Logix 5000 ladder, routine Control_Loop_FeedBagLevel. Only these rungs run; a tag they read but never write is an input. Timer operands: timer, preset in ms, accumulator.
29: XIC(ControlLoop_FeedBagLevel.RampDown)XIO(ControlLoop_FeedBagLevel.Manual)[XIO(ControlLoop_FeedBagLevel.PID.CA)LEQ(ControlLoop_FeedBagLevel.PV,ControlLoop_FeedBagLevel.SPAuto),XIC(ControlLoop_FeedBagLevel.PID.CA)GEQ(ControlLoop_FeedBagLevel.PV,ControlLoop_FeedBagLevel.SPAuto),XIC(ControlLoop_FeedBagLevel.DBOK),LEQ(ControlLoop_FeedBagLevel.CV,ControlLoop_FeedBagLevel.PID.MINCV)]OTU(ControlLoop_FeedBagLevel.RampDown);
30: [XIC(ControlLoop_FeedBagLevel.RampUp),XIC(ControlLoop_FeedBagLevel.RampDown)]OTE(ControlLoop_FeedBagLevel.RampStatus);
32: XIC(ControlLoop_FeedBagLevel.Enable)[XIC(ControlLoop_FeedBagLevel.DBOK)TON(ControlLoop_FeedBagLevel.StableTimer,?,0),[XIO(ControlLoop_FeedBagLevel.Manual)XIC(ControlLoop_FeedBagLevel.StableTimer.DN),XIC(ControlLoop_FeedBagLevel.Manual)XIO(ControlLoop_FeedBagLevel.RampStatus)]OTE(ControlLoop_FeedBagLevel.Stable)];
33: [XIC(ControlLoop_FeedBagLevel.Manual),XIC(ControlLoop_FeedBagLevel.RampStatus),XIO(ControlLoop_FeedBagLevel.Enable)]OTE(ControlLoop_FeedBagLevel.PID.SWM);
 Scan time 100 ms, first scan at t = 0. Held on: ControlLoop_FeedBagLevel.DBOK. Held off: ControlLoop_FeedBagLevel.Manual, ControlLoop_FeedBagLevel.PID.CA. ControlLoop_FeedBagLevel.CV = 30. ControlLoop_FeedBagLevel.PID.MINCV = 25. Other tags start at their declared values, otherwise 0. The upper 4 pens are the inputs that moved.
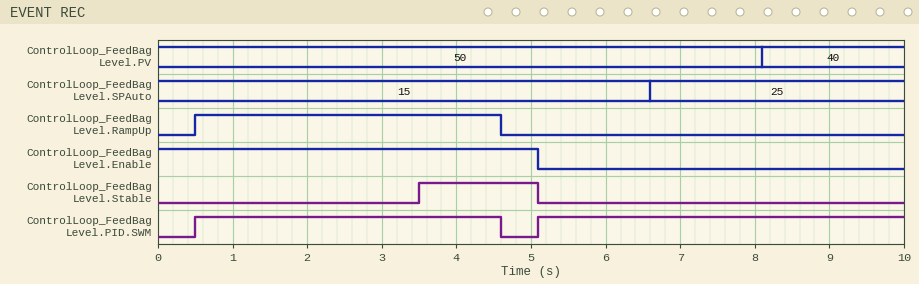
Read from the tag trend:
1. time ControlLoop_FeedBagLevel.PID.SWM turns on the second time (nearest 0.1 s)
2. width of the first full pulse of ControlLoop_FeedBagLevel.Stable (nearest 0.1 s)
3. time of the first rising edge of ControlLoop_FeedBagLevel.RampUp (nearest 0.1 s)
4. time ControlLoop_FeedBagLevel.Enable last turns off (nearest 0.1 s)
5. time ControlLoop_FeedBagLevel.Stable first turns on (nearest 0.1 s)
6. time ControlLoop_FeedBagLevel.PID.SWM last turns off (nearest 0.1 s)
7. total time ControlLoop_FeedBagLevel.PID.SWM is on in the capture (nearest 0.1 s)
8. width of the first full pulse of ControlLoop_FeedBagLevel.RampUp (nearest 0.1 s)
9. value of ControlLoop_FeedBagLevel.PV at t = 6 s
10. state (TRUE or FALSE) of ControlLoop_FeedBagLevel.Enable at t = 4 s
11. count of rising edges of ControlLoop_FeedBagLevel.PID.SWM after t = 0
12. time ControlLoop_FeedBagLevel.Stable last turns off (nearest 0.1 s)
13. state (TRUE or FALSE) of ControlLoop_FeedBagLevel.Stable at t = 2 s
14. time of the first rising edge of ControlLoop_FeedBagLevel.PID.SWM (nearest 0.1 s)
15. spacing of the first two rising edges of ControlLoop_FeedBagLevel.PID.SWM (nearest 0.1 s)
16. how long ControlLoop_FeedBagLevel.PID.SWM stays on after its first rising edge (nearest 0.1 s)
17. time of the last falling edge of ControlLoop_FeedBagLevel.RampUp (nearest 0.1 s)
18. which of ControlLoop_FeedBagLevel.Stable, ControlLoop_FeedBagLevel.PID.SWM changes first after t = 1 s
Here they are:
5.1 s
1.6 s
0.5 s
5.1 s
3.5 s
4.6 s
9.0 s
4.1 s
50
TRUE
2
5.1 s
FALSE
0.5 s
4.6 s
4.1 s
4.6 s
ControlLoop_FeedBagLevel.Stable
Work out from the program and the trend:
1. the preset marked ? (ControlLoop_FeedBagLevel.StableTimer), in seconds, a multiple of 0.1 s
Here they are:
3.5 s
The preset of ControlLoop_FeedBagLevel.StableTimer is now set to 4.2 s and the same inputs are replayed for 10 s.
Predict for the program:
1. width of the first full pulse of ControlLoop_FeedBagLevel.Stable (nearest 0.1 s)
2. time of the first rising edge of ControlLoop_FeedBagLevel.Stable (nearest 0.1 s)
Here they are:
0.9 s
4.2 s
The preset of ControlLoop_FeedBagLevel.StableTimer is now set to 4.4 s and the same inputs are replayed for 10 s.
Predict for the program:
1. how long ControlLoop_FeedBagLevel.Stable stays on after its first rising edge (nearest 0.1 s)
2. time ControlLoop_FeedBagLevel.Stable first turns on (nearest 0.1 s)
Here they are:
0.7 s
4.4 s
